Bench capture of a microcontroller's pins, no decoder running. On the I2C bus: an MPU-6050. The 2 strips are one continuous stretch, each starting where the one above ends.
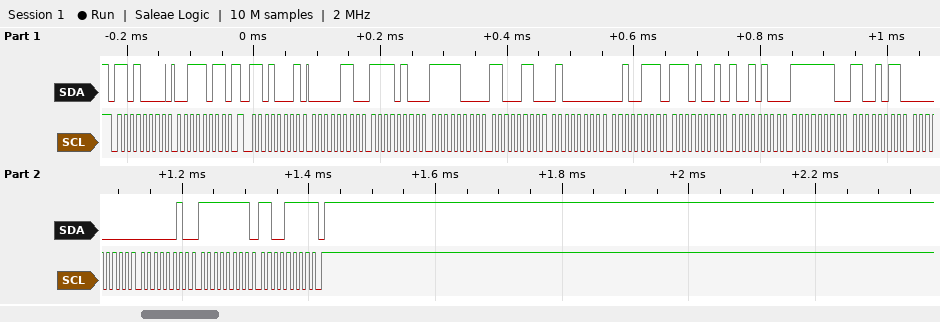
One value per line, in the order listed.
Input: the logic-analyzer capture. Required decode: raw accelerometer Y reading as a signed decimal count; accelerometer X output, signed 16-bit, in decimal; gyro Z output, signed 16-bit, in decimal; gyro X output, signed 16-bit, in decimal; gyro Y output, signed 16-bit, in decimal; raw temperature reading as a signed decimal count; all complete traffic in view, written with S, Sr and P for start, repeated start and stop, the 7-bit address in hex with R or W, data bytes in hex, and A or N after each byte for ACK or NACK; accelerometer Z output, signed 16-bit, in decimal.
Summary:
-1850
1780
-49
-309
2
-5740
S 68W A 3B A Sr 68R A 06 A F4 A F8 A C6 A 40 A 27 A E9 A 94 A FE A CB A 00 A 02 A FF A CF N P
16423
